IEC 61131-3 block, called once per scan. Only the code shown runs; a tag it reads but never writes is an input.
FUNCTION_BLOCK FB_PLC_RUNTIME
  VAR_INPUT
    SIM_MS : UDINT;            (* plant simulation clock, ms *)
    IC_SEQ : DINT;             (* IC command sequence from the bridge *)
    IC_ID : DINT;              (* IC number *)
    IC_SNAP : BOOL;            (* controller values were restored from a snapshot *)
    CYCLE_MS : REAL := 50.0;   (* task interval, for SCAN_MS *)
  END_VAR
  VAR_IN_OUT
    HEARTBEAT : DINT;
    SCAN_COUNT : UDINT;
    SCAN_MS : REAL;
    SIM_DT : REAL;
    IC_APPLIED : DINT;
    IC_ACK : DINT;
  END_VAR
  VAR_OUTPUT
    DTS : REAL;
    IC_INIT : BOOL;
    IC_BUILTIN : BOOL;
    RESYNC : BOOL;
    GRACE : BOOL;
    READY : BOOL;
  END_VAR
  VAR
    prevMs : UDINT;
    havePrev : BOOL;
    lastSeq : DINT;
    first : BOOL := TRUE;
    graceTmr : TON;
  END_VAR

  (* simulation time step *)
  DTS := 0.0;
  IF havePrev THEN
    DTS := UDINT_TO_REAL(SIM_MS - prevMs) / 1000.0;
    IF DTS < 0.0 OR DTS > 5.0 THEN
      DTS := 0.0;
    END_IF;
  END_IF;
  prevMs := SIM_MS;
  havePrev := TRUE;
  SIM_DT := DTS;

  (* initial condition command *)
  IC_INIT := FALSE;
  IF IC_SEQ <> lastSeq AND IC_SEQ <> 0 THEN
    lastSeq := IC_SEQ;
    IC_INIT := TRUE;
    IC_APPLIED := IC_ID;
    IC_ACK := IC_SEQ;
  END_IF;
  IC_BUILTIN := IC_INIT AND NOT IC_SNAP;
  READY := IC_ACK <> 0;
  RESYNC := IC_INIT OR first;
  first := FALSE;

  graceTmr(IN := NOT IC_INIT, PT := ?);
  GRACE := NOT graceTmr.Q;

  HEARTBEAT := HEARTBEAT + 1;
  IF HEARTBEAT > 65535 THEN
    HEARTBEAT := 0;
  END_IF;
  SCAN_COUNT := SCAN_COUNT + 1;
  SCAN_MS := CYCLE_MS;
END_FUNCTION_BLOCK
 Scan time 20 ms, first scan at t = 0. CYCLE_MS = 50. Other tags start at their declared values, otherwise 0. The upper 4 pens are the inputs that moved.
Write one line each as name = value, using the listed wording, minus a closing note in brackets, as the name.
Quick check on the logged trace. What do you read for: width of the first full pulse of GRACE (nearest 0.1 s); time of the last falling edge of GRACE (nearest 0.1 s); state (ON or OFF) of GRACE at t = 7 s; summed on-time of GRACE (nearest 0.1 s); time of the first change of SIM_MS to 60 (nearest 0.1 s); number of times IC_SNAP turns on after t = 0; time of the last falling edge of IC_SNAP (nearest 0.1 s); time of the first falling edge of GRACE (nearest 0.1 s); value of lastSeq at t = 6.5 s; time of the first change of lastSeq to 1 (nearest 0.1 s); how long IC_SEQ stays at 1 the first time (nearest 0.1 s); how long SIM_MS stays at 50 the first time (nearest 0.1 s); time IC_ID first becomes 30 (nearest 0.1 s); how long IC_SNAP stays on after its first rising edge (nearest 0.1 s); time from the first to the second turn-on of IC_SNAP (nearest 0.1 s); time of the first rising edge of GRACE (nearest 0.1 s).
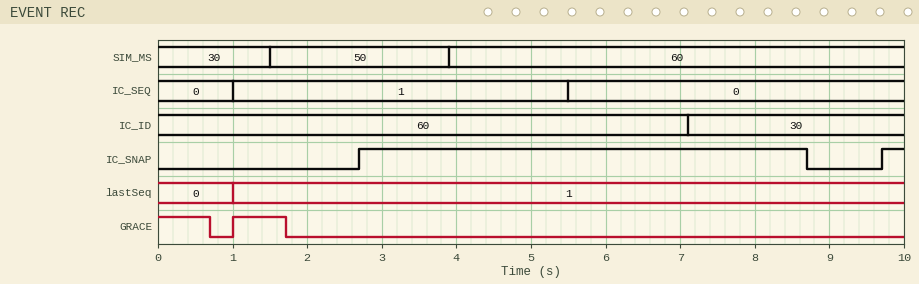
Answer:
width of the first full pulse of GRACE = 0.7 s
time of the last falling edge of GRACE = 1.7 s
state (ON or OFF) of GRACE at t = 7 s = OFF
summed on-time of GRACE = 1.4 s
time of the first change of SIM_MS to 60 = 3.9 s
number of times IC_SNAP turns on after t = 0 = 2
time of the last falling edge of IC_SNAP = 8.7 s
time of the first falling edge of GRACE = 0.7 s
value of lastSeq at t = 6.5 s = 1
time of the first change of lastSeq to 1 = 1.0 s
how long IC_SEQ stays at 1 the first time = 4.5 s
how long SIM_MS stays at 50 the first time = 2.4 s
time IC_ID first becomes 30 = 7.1 s
how long IC_SNAP stays on after its first rising edge = 6.0 s
time from the first to the second turn-on of IC_SNAP = 7.0 s
time of the first rising edge of GRACE = 1.0 s
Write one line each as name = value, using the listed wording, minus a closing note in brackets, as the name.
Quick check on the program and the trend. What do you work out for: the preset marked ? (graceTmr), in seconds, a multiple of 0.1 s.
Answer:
the preset marked ? (graceTmr), in seconds, a multiple of 0.1 s = 0.7 s
